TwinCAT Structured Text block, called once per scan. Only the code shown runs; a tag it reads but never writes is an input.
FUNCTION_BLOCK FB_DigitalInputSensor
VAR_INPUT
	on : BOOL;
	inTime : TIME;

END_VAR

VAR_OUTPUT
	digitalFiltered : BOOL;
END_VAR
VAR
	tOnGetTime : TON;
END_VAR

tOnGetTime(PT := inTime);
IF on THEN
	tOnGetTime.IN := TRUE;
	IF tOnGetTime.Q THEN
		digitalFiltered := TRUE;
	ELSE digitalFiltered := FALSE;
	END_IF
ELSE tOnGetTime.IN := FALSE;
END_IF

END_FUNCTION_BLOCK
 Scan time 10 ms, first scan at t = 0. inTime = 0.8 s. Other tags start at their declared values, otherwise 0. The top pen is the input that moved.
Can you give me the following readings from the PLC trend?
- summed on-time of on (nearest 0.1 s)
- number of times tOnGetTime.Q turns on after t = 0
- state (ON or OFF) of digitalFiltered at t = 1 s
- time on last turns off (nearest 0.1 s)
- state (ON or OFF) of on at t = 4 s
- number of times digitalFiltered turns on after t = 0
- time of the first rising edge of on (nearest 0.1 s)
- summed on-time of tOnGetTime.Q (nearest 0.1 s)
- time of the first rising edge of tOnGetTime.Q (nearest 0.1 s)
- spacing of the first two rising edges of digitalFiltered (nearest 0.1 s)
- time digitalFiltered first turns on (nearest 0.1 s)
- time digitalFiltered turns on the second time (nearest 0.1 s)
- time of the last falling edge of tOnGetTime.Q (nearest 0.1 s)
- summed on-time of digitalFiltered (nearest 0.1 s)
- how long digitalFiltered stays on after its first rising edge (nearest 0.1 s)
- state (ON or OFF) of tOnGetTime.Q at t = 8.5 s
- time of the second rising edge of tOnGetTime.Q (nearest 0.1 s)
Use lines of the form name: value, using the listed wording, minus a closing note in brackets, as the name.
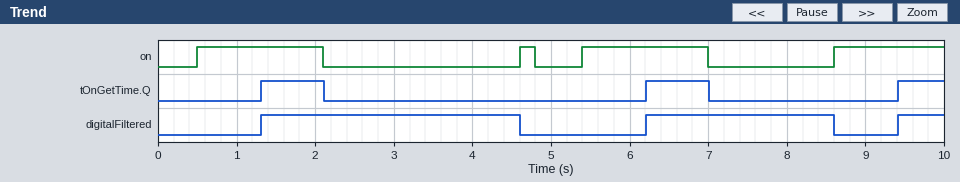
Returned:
summed on-time of on: 4.8 s
number of times tOnGetTime.Q turns on after t = 0: 3
state (ON or OFF) of digitalFiltered at t = 1 s: OFF
time on last turns off: 7.0 s
state (ON or OFF) of on at t = 4 s: OFF
number of times digitalFiltered turns on after t = 0: 3
time of the first rising edge of on: 0.5 s
summed on-time of tOnGetTime.Q: 2.2 s
time of the first rising edge of tOnGetTime.Q: 1.3 s
spacing of the first two rising edges of digitalFiltered: 4.9 s
time digitalFiltered first turns on: 1.3 s
time digitalFiltered turns on the second time: 6.2 s
time of the last falling edge of tOnGetTime.Q: 7.0 s
summed on-time of digitalFiltered: 6.3 s
how long digitalFiltered stays on after its first rising edge: 3.3 s
state (ON or OFF) of tOnGetTime.Q at t = 8.5 s: OFF
time of the second rising edge of tOnGetTime.Q: 6.2 s
